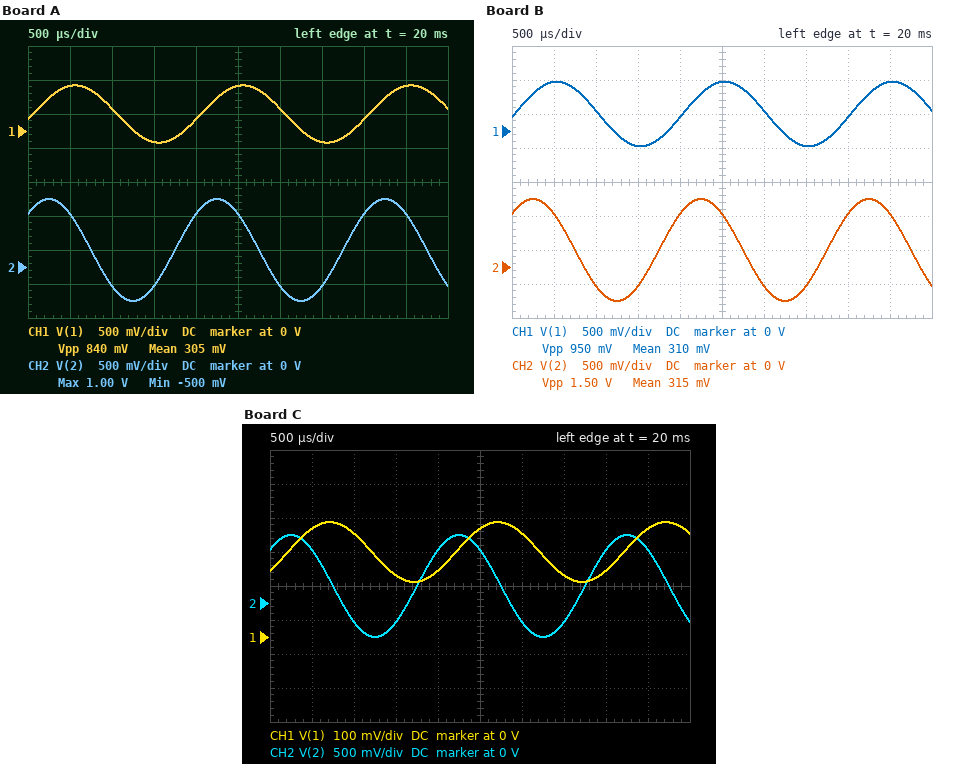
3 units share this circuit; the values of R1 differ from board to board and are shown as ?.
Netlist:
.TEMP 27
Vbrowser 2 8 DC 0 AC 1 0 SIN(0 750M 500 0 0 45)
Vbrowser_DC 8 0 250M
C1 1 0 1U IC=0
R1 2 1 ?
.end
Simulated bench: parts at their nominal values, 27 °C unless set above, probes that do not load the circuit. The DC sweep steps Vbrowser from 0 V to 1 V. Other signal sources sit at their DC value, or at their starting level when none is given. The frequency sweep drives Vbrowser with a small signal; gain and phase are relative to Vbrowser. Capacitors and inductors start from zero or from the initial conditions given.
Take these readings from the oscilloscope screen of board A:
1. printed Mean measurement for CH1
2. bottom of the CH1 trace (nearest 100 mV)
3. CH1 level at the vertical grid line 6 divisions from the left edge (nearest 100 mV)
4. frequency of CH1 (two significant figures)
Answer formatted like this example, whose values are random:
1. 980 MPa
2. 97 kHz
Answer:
1. 305 mV
2. -200 mV
3. 300 mV
4. 500 Hz
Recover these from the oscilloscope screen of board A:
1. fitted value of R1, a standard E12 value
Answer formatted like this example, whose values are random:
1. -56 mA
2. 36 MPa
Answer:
1. 470 Ω
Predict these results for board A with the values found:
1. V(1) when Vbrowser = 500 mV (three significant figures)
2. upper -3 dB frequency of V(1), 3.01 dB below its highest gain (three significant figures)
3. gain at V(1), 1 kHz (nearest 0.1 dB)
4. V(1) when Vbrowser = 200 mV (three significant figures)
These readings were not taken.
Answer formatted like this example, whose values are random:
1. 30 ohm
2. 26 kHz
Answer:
1. 750 mV
2. 339 Hz
3. -9.9 dB
4. 450 mV
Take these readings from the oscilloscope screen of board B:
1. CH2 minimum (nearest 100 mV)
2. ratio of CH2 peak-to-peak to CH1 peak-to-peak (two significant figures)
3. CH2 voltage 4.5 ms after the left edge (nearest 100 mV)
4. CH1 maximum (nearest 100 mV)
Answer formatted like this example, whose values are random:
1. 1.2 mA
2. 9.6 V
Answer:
1. -500 mV
2. 1.6
3. 800 mV
4. 700 mV
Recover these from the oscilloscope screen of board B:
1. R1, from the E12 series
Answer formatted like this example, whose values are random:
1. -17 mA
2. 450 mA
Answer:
1. 390 Ω
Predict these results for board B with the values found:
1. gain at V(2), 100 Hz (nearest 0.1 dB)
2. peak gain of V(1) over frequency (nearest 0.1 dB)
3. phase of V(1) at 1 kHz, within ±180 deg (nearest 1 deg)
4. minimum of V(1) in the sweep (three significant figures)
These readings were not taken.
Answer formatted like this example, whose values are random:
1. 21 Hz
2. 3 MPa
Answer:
1. 0 dB
2. 0 dB
3. -68 deg
4. 250 mV
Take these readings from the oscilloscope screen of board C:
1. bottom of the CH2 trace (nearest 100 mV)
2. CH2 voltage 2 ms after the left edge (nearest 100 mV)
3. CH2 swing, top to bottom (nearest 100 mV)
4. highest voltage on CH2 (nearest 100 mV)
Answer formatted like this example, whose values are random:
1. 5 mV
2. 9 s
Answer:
1. -500 mV
2. 800 mV
3. 1.5 V
4. 1.0 V
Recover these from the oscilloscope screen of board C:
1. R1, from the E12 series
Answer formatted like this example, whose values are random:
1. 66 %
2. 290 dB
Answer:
1. 2.7 kΩ
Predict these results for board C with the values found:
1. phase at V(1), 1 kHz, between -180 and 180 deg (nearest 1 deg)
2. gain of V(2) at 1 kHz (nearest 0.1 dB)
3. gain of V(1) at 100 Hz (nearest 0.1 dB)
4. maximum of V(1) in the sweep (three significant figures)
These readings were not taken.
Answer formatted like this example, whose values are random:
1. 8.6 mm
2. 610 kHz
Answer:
1. -87 deg
2. 0 dB
3. -5.9 dB
4. 1.25 V
